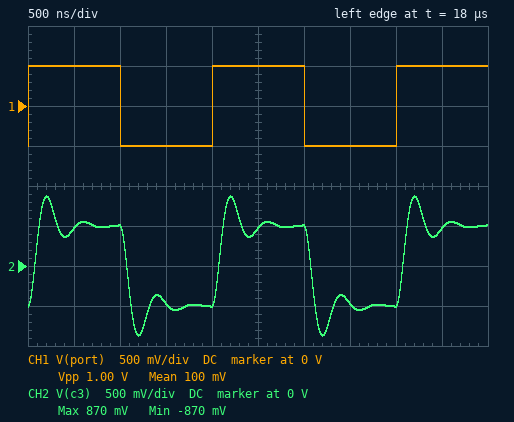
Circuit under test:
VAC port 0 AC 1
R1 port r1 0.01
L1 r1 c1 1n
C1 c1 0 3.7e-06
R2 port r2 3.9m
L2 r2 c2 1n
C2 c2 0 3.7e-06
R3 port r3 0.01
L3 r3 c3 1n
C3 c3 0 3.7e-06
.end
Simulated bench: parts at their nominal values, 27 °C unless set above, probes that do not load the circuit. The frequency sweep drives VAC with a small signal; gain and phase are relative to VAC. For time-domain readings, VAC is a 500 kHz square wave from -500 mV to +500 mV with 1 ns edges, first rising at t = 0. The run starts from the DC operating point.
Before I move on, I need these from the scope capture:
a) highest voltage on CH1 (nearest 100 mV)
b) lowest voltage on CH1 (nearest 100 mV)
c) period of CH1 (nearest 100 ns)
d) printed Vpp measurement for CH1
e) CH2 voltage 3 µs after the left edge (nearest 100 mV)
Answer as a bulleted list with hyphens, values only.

- 500 mV
- -500 mV
- 2.0 µs
- 1.00 V
- 500 mV
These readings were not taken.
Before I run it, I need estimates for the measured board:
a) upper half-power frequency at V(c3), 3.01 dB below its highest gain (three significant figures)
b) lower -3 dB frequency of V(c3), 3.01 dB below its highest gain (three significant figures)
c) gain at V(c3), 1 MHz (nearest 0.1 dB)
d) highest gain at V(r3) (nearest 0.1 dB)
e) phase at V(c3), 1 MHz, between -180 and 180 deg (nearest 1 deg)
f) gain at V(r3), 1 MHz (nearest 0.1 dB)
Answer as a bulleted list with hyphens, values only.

- 3.09 MHz
- 1.27 MHz
- 1.1 dB
- 0 dB
- -15 deg
- -0.3 dB
